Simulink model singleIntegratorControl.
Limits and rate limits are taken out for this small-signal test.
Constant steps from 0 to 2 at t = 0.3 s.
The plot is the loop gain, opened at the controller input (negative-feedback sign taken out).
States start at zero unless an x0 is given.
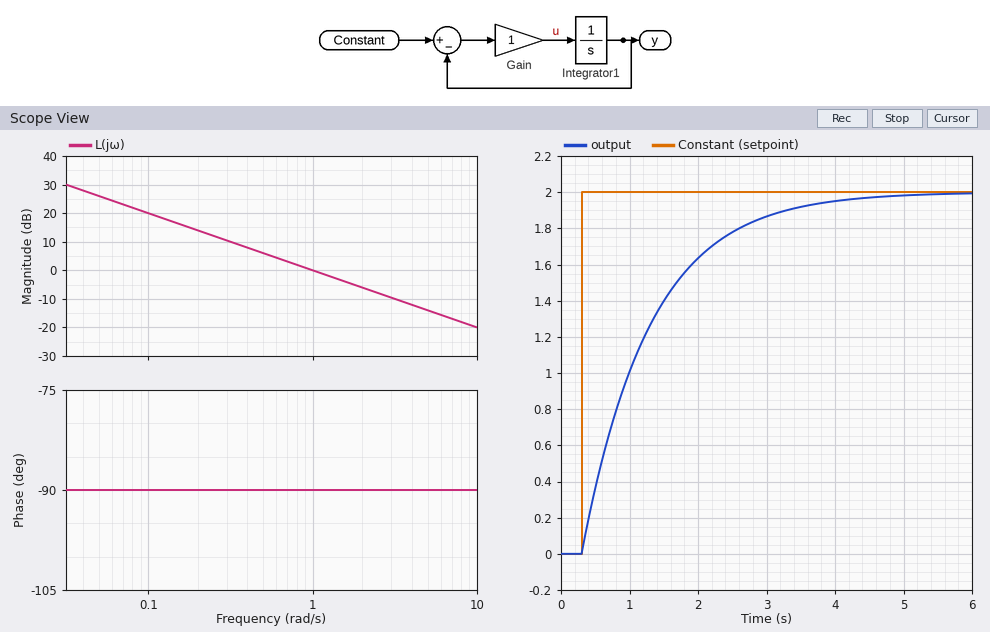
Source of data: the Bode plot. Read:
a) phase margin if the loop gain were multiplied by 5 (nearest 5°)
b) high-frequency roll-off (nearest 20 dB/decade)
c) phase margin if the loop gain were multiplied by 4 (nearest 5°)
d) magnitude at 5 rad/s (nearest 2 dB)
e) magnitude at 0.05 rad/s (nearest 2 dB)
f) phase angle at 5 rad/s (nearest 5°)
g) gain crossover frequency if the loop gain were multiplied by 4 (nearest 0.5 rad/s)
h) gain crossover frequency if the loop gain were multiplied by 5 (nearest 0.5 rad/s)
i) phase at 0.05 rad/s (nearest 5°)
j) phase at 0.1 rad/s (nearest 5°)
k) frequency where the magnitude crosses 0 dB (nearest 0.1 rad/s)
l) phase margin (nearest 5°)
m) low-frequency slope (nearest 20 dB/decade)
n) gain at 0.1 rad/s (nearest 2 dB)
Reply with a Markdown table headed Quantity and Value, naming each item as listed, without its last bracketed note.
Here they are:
| Quantity | Value |
|---|---|
| phase margin if the loop gain were multiplied by 5 | 90° |
| high-frequency roll-off | -20 dB/decade |
| phase margin if the loop gain were multiplied by 4 | 90° |
| magnitude at 5 rad/s | -14 dB |
| magnitude at 0.05 rad/s | 26 dB |
| phase angle at 5 rad/s | -90° |
| gain crossover frequency if the loop gain were multiplied by 4 | 4.0 rad/s |
| gain crossover frequency if the loop gain were multiplied by 5 | 5.0 rad/s |
| phase at 0.05 rad/s | -90° |
| phase at 0.1 rad/s | -90° |
| frequency where the magnitude crosses 0 dB | 1.0 rad/s |
| phase margin | 90° |
| low-frequency slope | -20 dB/decade |
| gain at 0.1 rad/s | 20 dB |
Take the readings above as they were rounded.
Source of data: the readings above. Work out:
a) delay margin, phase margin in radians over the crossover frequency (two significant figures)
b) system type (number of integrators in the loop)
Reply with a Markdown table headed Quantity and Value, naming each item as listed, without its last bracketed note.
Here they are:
| Quantity | Value |
|---|---|
| delay margin, phase margin in radians over the crossover frequency | 1.6 s |
| system type | 1 |
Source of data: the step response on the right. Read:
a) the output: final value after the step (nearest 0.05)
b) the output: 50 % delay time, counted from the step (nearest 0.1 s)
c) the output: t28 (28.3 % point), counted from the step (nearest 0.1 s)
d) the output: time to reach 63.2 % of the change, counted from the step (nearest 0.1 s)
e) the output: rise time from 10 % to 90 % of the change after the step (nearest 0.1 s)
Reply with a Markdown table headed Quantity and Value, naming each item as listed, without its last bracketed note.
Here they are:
| Quantity | Value |
|---|---|
| the output: final value after the step | 2.00 |
| the output: 50 % delay time, counted from the step | 0.7 s |
| the output: t28 (28.3 % point), counted from the step | 0.3 s |
| the output: time to reach 63.2 % of the change, counted from the step | 1.0 s |
| the output: rise time from 10 % to 90 % of the change after the step | 2.2 s |
